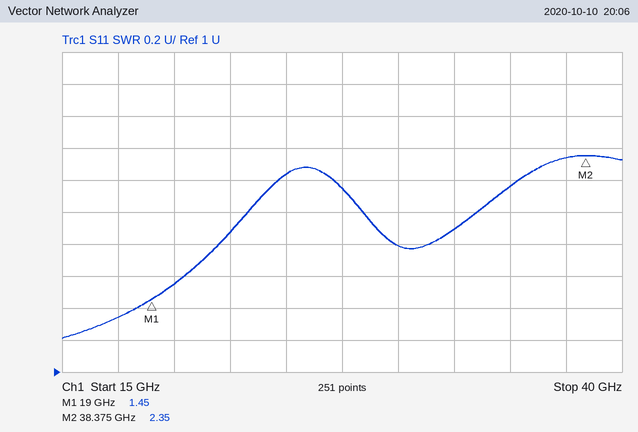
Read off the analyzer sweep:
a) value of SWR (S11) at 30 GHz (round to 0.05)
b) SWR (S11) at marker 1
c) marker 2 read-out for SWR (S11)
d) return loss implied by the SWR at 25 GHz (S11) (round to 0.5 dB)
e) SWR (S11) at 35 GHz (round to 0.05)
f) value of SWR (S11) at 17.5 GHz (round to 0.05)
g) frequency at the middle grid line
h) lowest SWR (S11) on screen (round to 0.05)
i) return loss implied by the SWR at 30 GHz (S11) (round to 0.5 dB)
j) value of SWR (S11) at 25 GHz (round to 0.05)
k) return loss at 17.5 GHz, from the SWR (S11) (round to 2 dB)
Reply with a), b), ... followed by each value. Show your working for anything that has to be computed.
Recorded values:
a) 1.80
b) 1.45
c) 2.35
d) −20 log10((2.25 − 1)/(2.25 + 1)) ≈ 8.30 dB, so 8.5 dB to the nearest 0.5 dB
e) 2.15
f) 1.35
g) 27.5 GHz
h) 1.20
i) −20 log10((1.8 − 1)/(1.8 + 1)) ≈ 10.9 dB, so 11.0 dB to the nearest 0.5 dB
j) 2.25
k) −20 log10((1.35 − 1)/(1.35 + 1)) ≈ 16 dB
